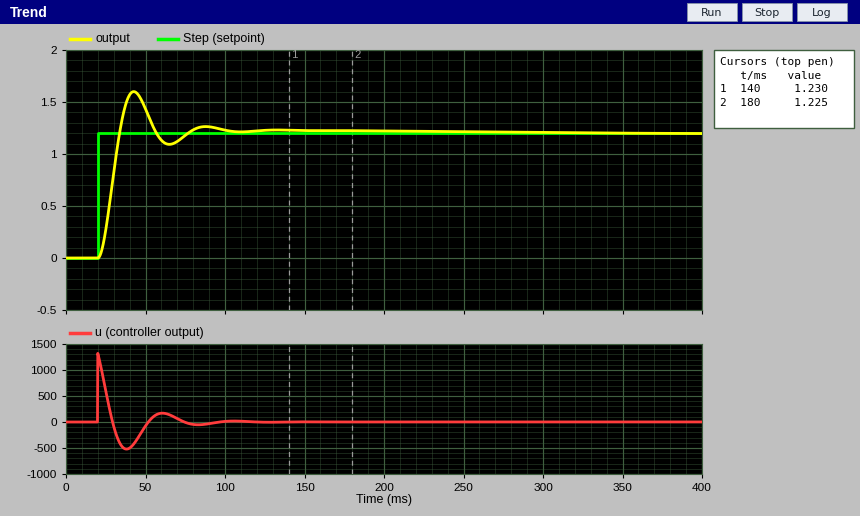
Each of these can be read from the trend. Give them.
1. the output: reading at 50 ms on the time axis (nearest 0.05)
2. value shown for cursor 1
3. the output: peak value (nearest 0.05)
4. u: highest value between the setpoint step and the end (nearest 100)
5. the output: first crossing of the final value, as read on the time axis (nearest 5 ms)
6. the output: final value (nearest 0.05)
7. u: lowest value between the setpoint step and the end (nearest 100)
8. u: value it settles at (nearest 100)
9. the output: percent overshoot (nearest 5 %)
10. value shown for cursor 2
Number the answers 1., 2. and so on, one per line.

1. 1.45
2. 1.230
3. 1.60
4. 1300
5. 35 ms
6. 1.20
7. -500
8. 0
9. 35 %
10. 1.225
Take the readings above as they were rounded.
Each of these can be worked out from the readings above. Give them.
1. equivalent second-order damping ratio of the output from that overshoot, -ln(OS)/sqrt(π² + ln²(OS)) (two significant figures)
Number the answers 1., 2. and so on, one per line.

1. 0.32
